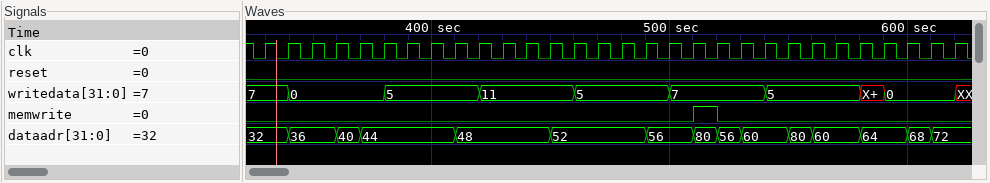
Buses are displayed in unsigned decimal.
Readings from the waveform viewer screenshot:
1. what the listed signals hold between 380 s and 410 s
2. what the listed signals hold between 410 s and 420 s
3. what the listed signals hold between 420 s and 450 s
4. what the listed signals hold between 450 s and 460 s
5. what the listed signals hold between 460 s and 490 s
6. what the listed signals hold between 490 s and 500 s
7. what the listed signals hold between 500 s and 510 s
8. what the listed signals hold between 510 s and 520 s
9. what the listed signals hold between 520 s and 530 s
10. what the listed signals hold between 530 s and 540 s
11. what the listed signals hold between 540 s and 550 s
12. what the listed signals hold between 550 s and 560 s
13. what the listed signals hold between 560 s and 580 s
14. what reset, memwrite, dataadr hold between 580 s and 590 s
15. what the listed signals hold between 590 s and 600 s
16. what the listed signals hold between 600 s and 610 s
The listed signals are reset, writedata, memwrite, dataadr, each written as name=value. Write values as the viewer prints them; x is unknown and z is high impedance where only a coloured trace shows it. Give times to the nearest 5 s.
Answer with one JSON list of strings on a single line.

["reset=0, writedata=5, memwrite=0, dataadr=44", "reset=0, writedata=5, memwrite=0, dataadr=48", "reset=0, writedata=11, memwrite=0, dataadr=48", "reset=0, writedata=11, memwrite=0, dataadr=52", "reset=0, writedata=5, memwrite=0, dataadr=52", "reset=0, writedata=5, memwrite=0, dataadr=56", "reset=0, writedata=7, memwrite=0, dataadr=56", "reset=0, writedata=7, memwrite=1, dataadr=80", "reset=0, writedata=7, memwrite=0, dataadr=56", "reset=0, writedata=7, memwrite=0, dataadr=60", "reset=0, writedata=5, memwrite=0, dataadr=60", "reset=0, writedata=5, memwrite=0, dataadr=80", "reset=0, writedata=5, memwrite=0, dataadr=60", "reset=0, memwrite=0, dataadr=64", "reset=0, writedata=0, memwrite=0, dataadr=64", "reset=0, writedata=0, memwrite=0, dataadr=68"]
